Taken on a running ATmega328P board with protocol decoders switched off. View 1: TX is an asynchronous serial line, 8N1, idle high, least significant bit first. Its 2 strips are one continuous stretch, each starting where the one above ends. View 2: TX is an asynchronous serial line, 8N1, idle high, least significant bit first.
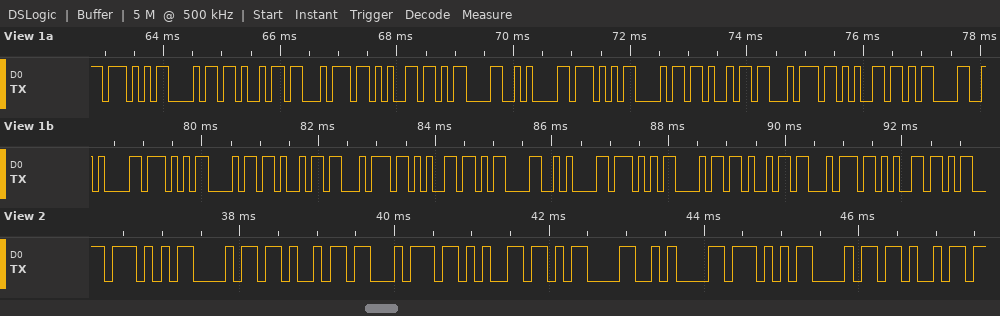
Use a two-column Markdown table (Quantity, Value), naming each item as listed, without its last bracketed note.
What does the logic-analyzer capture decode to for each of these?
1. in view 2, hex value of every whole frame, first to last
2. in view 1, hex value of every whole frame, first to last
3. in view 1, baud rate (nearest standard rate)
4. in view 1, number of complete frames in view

| Quantity | Value |
|---|---|
| in view 2, hex value of every whole frame, first to last | 57 68 69 74 65 0D 0A 57 68 69 |
| in view 1, hex value of every whole frame, first to last | 0x57 0x68 0x69 0x74 0x65 0x0D 0x0A 0x57 0x68 0x69 0x74 0x65 0x0D 0x0A 0x57 0x68 0x69 0x74 0x65 0x0D 0x0A 0x57 0x68 0x69 0x74 0x65 |
| in view 1, baud rate | 9600 baud |
| in view 1, number of complete frames in view | 26 |
